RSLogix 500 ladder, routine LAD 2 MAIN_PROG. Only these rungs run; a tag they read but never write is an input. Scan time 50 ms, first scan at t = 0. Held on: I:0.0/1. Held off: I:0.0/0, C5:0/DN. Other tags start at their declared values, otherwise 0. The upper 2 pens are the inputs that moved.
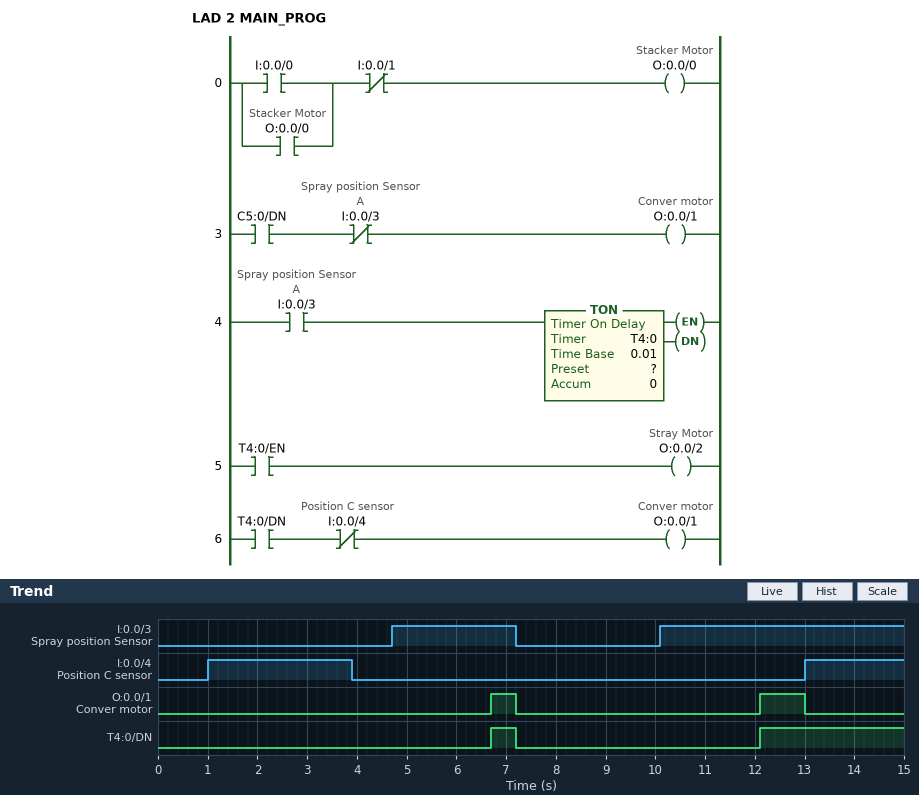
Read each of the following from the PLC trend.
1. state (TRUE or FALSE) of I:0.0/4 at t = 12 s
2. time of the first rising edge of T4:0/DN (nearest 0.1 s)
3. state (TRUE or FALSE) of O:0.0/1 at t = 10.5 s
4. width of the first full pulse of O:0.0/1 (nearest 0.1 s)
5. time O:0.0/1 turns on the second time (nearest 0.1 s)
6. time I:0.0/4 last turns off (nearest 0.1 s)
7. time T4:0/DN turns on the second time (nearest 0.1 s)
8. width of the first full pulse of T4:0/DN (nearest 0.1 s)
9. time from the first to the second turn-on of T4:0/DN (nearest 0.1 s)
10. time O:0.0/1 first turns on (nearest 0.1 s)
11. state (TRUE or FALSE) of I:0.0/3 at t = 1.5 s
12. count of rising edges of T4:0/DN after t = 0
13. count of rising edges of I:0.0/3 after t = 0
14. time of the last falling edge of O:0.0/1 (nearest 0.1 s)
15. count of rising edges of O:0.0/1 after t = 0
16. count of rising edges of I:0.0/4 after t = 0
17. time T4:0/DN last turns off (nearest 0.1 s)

FALSE
6.7 s
FALSE
0.5 s
12.1 s
3.9 s
12.1 s
0.5 s
5.4 s
6.7 s
FALSE
2
2
13.0 s
2
2
7.2 s
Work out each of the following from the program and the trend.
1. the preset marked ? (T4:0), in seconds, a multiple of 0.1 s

2.0 s
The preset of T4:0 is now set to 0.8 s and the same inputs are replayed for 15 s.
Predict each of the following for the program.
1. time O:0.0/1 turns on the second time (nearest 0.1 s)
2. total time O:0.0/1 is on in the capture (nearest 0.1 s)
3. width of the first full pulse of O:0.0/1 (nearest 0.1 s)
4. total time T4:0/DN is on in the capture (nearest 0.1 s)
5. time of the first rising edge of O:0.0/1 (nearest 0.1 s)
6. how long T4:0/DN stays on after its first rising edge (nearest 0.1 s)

10.9 s
3.8 s
1.7 s
5.8 s
5.5 s
1.7 s
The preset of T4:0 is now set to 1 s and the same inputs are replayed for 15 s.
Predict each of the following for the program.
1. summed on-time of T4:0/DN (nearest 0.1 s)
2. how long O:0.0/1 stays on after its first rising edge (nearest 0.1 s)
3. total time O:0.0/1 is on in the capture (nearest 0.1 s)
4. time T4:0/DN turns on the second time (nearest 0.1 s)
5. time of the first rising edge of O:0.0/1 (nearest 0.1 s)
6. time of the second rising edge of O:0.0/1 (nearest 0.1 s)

5.4 s
1.5 s
3.4 s
11.1 s
5.7 s
11.1 s
